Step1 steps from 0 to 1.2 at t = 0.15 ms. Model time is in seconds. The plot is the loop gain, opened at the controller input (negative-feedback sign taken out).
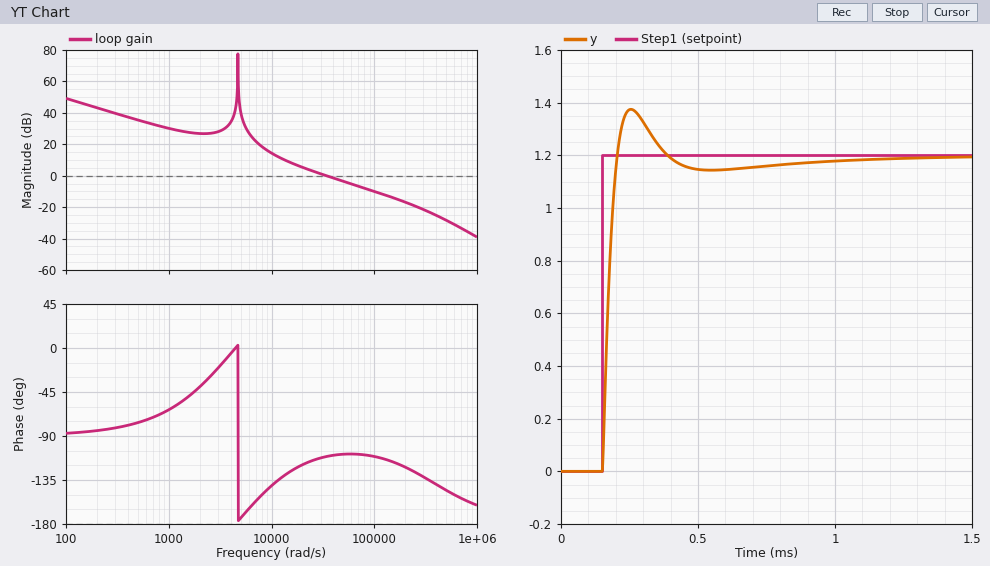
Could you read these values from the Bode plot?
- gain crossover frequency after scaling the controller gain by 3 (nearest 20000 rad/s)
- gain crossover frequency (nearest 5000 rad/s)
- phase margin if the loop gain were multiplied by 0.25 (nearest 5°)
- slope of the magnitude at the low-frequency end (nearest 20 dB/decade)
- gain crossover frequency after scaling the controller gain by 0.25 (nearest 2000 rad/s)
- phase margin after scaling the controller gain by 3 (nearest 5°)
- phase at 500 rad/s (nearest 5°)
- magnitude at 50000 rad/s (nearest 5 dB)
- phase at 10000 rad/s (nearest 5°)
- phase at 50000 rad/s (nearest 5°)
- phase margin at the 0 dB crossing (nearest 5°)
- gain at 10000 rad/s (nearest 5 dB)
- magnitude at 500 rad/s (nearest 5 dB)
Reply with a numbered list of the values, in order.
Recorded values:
1. 100000 rad/s
2. 35000 rad/s
3. 45°
4. -20 dB/decade
5. 12000 rad/s
6. 70°
7. -75°
8. -5 dB
9. -140°
10. -110°
11. 70°
12. 15 dB
13. 35 dB
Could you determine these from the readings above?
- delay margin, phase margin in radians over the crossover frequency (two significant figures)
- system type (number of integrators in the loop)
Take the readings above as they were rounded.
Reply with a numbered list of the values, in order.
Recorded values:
1. 0.000035 s
2. 1
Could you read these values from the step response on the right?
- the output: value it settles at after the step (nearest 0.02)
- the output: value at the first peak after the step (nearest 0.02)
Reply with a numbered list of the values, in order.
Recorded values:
1. 1.20
2. 1.38
